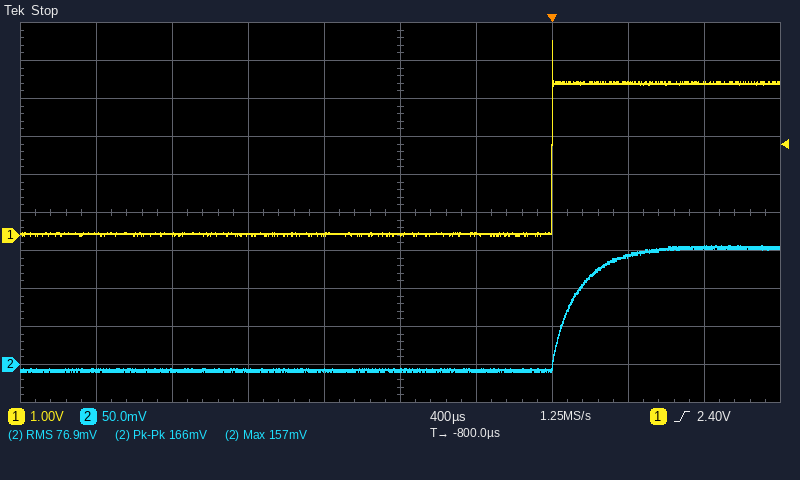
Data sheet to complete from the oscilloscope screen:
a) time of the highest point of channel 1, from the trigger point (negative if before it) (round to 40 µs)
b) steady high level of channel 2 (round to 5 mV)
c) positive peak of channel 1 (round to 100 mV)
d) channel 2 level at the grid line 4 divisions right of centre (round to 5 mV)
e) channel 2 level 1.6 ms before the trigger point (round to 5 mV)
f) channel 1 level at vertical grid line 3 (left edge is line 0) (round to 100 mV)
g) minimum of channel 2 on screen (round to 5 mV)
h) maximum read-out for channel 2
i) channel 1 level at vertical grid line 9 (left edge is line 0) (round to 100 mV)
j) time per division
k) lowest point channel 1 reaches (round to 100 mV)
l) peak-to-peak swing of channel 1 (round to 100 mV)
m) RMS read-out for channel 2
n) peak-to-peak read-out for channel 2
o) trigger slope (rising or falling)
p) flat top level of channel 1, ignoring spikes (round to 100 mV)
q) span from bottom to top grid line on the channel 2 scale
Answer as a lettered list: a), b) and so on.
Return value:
a) 0 µs
b) 155 mV
c) 5.1 V
d) 155 mV
e) -5 mV
f) 0.0 V
g) -10 mV
h) 157 mV
i) 4.0 V
j) 400 µs
k) 0.0 V
l) 5.1 V
m) 76.9 mV
n) 166 mV
o) rising
p) 4.0 V
q) 500 mV
